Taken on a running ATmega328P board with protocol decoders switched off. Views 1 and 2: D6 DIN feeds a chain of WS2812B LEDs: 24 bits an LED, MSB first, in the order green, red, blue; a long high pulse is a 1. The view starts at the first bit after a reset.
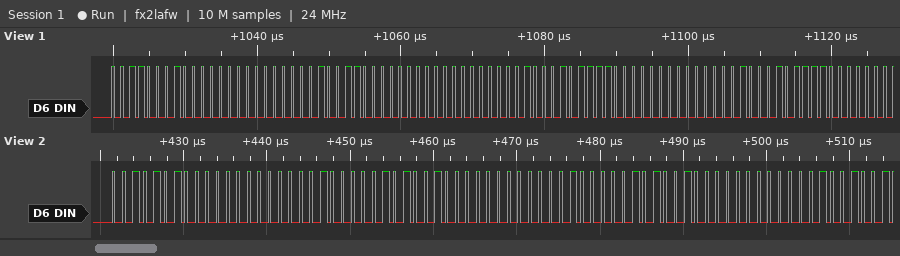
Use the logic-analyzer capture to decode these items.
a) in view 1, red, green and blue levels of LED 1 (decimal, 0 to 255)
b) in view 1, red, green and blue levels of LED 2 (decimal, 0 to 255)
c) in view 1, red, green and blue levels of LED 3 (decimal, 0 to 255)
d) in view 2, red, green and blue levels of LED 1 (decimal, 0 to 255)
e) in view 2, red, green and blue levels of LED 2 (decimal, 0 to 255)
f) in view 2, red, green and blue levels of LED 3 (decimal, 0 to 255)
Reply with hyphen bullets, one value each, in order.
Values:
- 0, 49, 1
- 0, 48, 2
- 0, 47, 2
- 0, 42, 8
- 0, 41, 8
- 0, 41, 9
